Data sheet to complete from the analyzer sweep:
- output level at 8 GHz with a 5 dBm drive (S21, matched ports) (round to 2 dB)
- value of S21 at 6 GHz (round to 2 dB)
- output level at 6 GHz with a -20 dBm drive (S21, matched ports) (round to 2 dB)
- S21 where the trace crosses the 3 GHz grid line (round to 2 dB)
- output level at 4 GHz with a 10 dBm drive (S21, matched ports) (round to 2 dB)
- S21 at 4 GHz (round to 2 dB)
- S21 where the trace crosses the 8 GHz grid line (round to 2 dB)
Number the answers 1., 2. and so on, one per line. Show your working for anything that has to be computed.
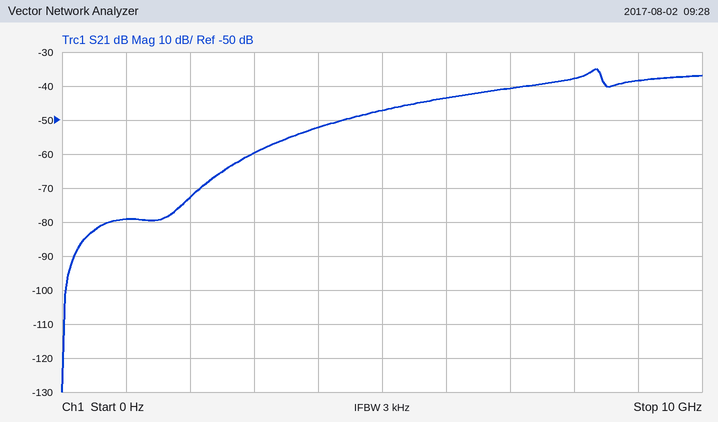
1. 5 dBm + (-38 dB) = -32 dBm
2. -44 dB
3. -20 dBm + (-44 dB) = -64 dBm
4. -60 dB
5. 10 dBm + (-52 dB) = -42 dBm
6. -52 dB
7. -38 dB
